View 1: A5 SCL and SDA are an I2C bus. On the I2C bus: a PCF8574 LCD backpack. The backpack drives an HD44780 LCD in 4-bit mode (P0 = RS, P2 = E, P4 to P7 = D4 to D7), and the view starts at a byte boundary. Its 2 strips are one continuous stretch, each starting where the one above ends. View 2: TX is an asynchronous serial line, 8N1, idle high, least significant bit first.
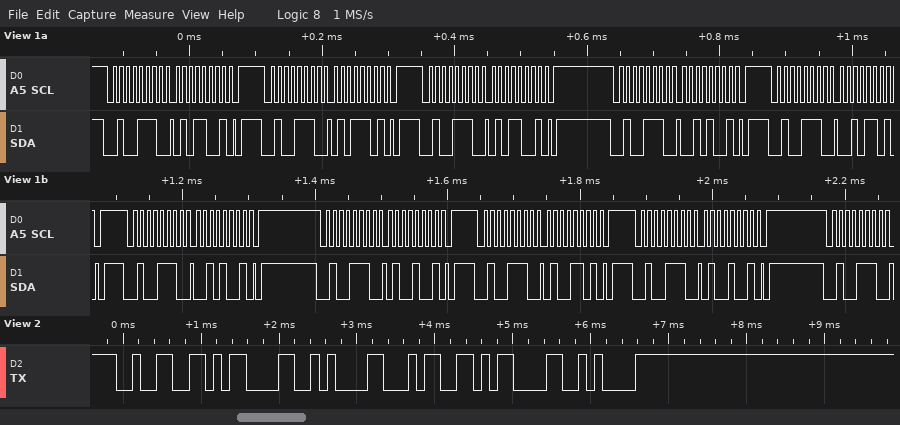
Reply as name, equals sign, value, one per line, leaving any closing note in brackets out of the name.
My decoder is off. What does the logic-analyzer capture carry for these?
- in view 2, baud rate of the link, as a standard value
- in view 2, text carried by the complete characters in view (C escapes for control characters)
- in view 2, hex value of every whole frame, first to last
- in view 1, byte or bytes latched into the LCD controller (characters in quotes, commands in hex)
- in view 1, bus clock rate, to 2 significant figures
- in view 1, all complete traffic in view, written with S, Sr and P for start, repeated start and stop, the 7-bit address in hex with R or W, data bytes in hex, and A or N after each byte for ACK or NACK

in view 2, baud rate of the link, as a standard value = 9600 baud
in view 2, text carried by the complete characters in view = "2\r\n4\r\n"
in view 2, hex value of every whole frame, first to last = 32 0D 0A 34 0D 0A
in view 1, byte or bytes latched into the LCD controller = 'R'
in view 1, bus clock rate, to 2 significant figures = 100 kHz
in view 1, all complete traffic in view, written with S, Sr and P for start, repeated start and stop, the 7-bit address in hex with R or W, data bytes in hex, and A or N after each byte for ACK or NACK = S 27W A 59 A P S 27W A 5D A P S 27W A 59 A P S 27W A 29 A P S 27W A 2D A P S 27W A 29 A P S 27W A 49 A P S 27W A 4D A P S 27W A 49 A P S 27W A
